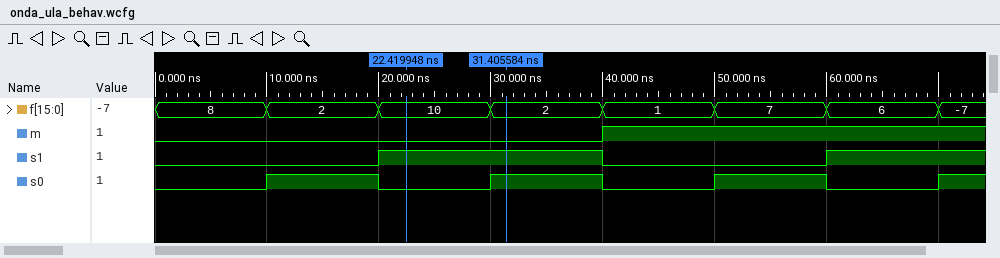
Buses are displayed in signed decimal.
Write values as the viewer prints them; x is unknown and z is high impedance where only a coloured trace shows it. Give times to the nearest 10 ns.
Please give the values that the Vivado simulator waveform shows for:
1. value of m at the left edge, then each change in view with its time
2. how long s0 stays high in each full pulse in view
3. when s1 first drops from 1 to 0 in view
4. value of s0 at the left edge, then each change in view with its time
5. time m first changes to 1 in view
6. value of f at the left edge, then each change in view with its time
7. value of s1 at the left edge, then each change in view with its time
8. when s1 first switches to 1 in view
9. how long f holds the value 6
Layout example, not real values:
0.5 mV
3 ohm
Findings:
0, 1 at 40 ns
10 ns, 10 ns, 10 ns
40 ns
0, 1 at 10 ns, 0 at 20 ns, 1 at 30 ns, 0 at 40 ns, 1 at 50 ns, 0 at 60 ns, 1 at 70 ns
40 ns
8, 2 at 10 ns, 10 at 20 ns, 2 at 30 ns, 1 at 40 ns, 7 at 50 ns, 6 at 60 ns, -7 at 70 ns
0, 1 at 20 ns, 0 at 40 ns, 1 at 60 ns
20 ns
10 ns
